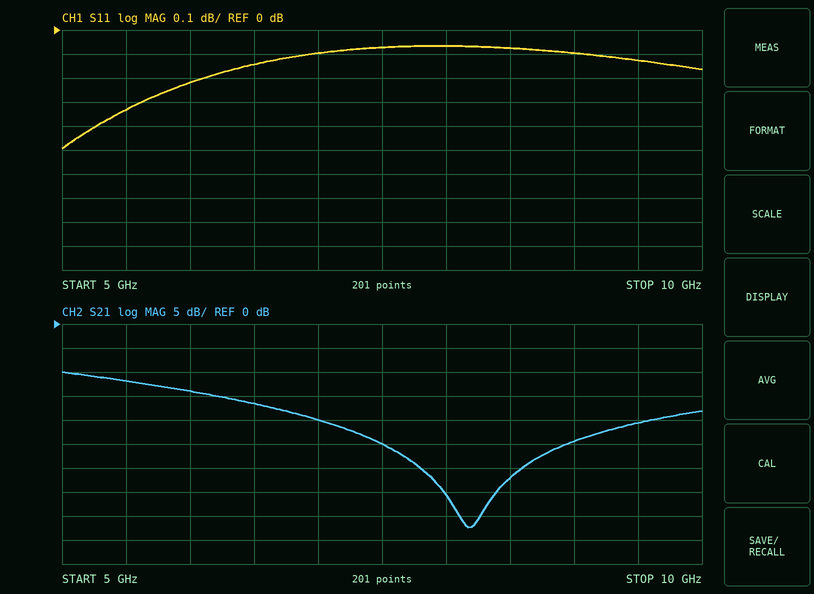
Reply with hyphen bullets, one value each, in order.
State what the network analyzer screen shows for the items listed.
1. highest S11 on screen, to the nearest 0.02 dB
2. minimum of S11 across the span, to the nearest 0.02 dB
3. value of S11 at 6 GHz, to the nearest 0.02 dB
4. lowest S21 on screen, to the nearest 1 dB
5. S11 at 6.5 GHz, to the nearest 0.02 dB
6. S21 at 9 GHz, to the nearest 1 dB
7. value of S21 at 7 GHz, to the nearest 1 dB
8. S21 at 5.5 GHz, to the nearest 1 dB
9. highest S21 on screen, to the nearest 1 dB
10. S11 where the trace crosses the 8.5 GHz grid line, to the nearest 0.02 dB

- -0.06 dB
- -0.50 dB
- -0.22 dB
- -42 dB
- -0.14 dB
- -24 dB
- -20 dB
- -12 dB
- -10 dB
- -0.08 dB
